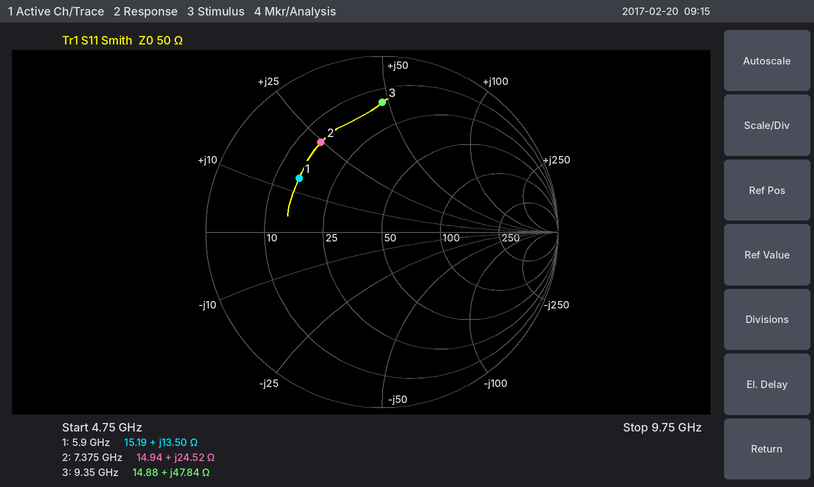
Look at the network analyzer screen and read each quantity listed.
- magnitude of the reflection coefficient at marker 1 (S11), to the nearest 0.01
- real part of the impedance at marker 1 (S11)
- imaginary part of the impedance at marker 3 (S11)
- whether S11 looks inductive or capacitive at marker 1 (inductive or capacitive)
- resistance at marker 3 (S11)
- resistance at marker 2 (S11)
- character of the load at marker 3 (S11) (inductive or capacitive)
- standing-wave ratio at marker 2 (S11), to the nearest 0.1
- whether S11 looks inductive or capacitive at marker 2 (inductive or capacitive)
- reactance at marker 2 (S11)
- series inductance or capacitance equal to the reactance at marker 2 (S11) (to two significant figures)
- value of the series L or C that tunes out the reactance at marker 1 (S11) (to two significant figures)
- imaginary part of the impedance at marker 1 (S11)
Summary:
0.56
15.19 Ω
+47.84 Ω
inductive
14.88 Ω
14.94 Ω
inductive
4.2
inductive
+24.52 Ω
530 pH
2.0 pF
+13.50 Ω
